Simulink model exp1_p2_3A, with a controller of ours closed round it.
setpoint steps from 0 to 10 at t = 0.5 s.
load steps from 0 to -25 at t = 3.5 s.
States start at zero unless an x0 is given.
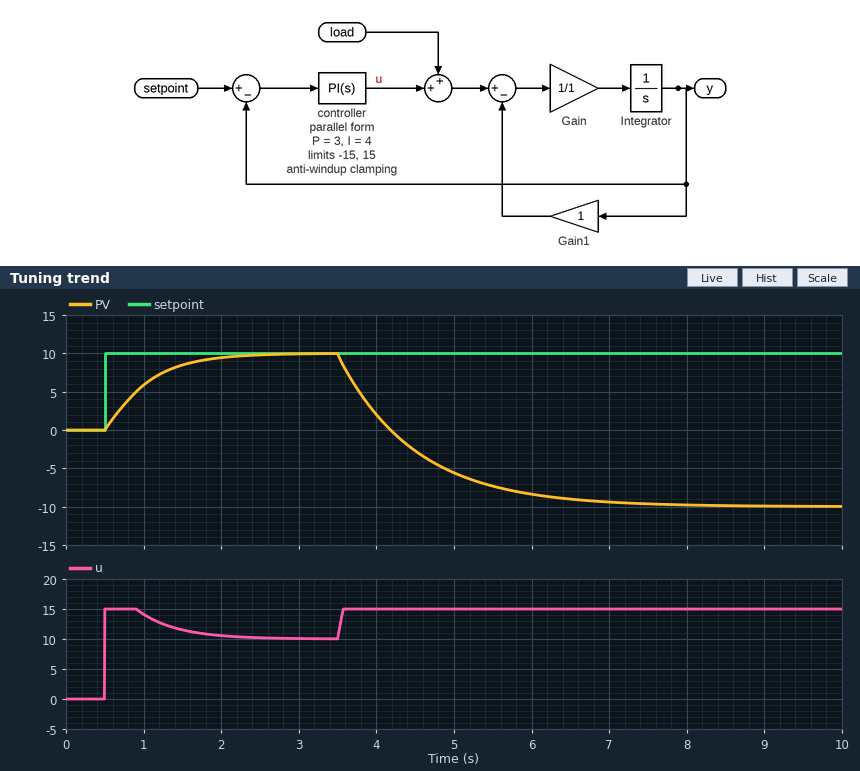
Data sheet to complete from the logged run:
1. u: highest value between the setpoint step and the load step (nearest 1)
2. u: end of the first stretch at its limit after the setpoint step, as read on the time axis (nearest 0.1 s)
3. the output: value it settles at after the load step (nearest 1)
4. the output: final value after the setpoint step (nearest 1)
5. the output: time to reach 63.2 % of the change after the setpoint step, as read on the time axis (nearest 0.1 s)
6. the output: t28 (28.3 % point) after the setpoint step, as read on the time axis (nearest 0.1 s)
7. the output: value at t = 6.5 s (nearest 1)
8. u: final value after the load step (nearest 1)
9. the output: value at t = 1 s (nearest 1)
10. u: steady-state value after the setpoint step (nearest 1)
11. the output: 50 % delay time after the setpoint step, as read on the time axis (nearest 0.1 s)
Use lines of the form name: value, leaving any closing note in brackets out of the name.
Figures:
u: highest value between the setpoint step and the load step: 15
u: end of the first stretch at its limit after the setpoint step, as read on the time axis: 0.9 s
the output: value it settles at after the load step: -10
the output: final value after the setpoint step: 10
the output: time to reach 63.2 % of the change after the setpoint step, as read on the time axis: 1.1 s
the output: t28 (28.3 % point) after the setpoint step, as read on the time axis: 0.7 s
the output: value at t = 6.5 s: -9
u: final value after the load step: 15
the output: value at t = 1 s: 6
u: steady-state value after the setpoint step: 10
the output: 50 % delay time after the setpoint step, as read on the time axis: 0.9 s
